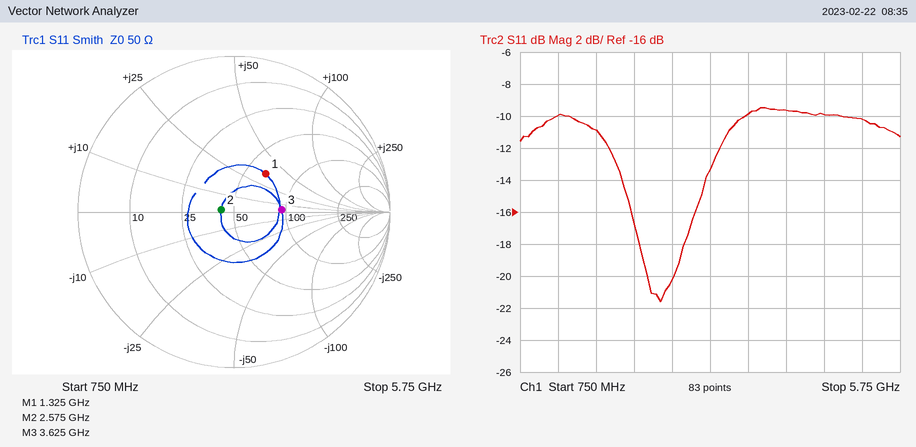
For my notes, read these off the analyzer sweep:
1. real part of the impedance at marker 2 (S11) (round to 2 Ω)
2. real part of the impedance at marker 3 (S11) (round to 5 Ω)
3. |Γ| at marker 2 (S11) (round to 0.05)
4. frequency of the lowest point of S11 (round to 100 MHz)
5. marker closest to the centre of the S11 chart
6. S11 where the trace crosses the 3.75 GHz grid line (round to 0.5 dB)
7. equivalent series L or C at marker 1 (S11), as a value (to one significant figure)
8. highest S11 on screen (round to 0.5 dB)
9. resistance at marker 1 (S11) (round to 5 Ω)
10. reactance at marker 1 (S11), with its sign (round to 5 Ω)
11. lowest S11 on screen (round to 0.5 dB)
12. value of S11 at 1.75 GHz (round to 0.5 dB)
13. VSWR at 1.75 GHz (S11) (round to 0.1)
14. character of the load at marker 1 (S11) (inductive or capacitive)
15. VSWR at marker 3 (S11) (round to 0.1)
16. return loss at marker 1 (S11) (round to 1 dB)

42 Ω
95 Ω
0.10
2.6 GHz
marker 2
-10.0 dB
4 nH
-9.5 dB
65 Ω
+35 Ω
-21.5 dB
-11.0 dB
1.8
inductive
1.9
10 dB
